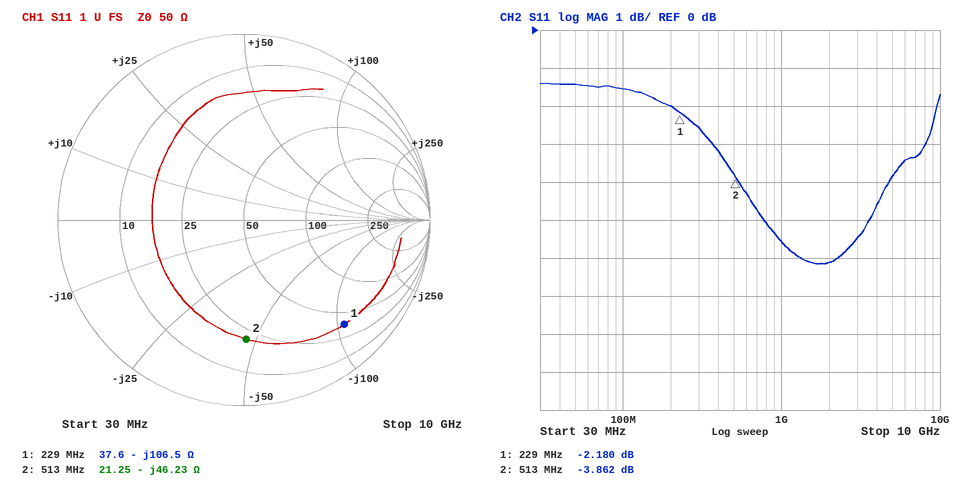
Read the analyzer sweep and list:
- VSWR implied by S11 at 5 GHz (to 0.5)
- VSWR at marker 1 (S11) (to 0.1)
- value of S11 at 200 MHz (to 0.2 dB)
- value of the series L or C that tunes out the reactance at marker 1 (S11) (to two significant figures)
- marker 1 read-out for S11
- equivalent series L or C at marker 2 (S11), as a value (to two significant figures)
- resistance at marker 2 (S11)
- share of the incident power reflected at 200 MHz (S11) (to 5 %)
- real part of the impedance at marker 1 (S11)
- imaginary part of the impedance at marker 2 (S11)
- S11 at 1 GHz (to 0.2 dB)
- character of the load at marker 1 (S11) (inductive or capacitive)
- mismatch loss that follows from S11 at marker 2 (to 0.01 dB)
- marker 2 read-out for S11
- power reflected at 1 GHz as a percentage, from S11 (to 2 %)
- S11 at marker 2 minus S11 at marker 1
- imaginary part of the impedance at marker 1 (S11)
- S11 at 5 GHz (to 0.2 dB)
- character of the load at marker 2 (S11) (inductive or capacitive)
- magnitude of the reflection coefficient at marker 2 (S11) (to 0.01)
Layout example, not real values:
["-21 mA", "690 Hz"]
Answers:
["4.5", "8.0", "-2.0 dB", "74 nH", "-2.180 dB", "6.7 pF", "21.25 Ω", "65 %", "37.6 Ω", "-46.23 Ω", "-5.6 dB", "capacitive", "2.30 dB", "-3.862 dB", "28 %", "-1.682 dB", "-106.5 Ω", "-3.8 dB", "capacitive", "0.64"]
